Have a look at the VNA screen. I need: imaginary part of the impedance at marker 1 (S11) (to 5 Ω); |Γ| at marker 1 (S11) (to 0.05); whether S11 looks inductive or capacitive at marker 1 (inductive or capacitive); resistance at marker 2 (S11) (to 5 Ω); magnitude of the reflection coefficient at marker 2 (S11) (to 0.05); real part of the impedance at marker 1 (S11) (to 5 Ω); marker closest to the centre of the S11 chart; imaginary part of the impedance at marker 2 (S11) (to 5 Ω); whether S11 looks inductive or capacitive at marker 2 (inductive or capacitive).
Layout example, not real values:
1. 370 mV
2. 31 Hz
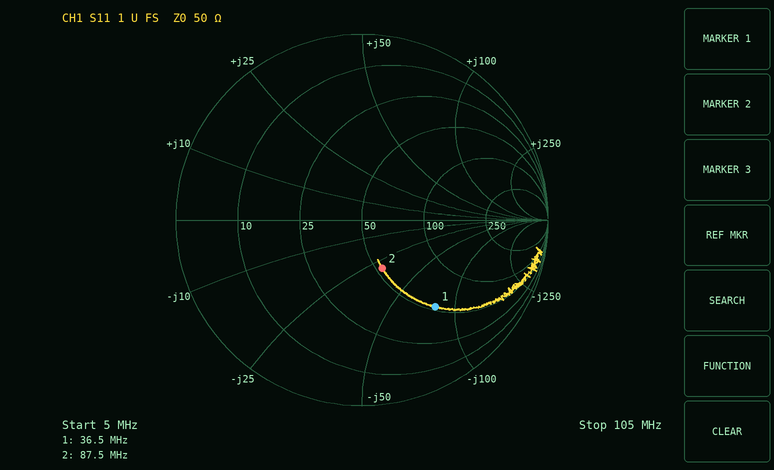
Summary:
1. -80 Ω
2. 0.60
3. capacitive
4. 55 Ω
5. 0.30
6. 55 Ω
7. marker 2
8. -30 Ω
9. capacitive
